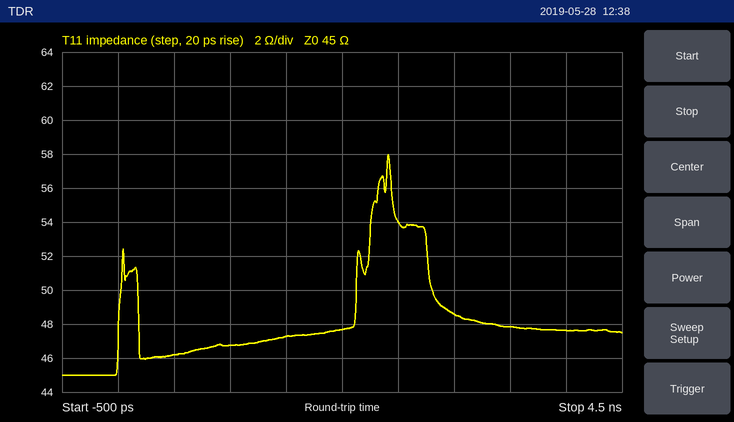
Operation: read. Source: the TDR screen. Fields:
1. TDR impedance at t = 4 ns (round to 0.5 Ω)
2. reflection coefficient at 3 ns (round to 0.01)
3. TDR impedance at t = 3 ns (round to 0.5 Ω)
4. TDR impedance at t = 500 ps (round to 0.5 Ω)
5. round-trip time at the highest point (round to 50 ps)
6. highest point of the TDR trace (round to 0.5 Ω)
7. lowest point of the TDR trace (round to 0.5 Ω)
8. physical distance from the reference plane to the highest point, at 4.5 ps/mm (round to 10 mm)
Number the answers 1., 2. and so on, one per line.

1. 47.5 Ω
2. +0.04
3. 48.5 Ω
4. 46.0 Ω
5. 2.40 ns
6. 58.0 Ω
7. 45.0 Ω
8. 270 mm
